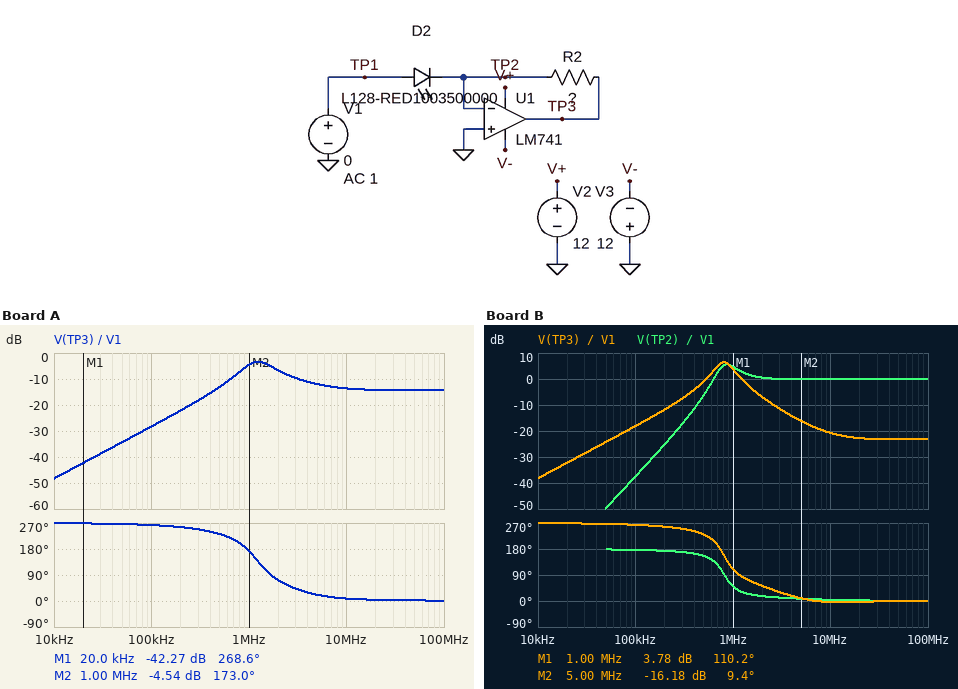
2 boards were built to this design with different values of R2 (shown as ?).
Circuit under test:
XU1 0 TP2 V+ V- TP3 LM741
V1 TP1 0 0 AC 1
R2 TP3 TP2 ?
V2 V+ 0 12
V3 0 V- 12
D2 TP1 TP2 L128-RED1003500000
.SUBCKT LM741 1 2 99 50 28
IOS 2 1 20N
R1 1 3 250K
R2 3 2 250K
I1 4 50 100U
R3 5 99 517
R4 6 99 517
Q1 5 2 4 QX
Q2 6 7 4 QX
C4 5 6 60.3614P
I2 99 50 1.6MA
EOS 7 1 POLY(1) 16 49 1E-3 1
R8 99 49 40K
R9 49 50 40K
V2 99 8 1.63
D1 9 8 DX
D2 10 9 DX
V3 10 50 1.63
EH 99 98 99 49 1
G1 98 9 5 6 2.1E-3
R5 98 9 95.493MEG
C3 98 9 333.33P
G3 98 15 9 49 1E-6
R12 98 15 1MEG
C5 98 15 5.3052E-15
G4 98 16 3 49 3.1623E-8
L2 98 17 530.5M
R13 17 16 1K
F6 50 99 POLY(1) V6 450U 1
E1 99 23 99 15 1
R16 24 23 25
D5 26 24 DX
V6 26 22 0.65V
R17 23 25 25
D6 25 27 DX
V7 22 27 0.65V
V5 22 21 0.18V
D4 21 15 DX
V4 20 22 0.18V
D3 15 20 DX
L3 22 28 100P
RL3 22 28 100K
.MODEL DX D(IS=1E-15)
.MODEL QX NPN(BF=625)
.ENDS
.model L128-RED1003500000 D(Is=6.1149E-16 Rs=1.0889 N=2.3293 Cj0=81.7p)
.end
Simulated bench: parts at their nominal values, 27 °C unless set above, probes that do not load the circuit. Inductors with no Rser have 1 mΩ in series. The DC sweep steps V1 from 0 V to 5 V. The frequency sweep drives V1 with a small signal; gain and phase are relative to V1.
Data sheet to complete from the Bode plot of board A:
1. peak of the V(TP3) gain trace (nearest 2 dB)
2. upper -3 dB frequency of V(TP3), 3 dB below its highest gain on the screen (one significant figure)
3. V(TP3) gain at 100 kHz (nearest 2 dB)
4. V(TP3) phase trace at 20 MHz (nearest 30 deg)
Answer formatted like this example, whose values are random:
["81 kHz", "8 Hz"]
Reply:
["-4 dB", "2 MHz", "-28 dB", "0 deg"]
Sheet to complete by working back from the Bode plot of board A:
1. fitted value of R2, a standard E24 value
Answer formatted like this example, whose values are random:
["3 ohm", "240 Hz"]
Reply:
["750 Ω"]
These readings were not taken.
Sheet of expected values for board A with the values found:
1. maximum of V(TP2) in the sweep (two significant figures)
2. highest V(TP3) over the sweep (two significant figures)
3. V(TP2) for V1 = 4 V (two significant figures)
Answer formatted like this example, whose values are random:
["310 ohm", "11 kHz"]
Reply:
["3.1 V", "1.1 mV", "2.1 V"]
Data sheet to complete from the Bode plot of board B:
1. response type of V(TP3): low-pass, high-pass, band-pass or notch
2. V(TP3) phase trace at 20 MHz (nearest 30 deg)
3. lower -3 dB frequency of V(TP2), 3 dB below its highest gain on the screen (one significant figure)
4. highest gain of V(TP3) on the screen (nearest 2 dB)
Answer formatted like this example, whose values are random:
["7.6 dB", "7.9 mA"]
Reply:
["band-pass", "0 deg", "700 kHz", "6 dB"]
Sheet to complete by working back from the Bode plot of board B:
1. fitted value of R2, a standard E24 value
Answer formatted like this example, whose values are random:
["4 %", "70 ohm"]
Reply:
["2.4 kΩ"]
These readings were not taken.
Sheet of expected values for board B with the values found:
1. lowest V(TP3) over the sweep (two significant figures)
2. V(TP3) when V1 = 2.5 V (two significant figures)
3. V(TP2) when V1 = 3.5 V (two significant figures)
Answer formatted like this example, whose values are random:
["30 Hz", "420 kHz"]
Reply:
["-11 V", "-11 V", "1.7 V"]
